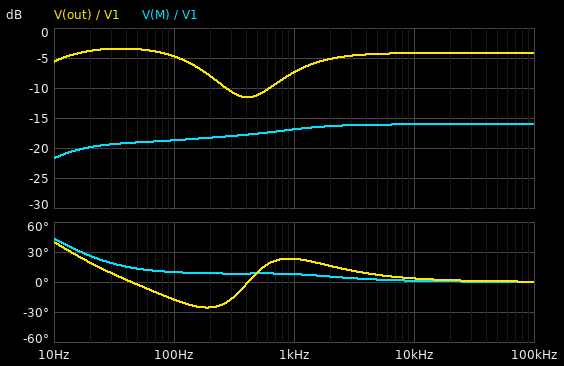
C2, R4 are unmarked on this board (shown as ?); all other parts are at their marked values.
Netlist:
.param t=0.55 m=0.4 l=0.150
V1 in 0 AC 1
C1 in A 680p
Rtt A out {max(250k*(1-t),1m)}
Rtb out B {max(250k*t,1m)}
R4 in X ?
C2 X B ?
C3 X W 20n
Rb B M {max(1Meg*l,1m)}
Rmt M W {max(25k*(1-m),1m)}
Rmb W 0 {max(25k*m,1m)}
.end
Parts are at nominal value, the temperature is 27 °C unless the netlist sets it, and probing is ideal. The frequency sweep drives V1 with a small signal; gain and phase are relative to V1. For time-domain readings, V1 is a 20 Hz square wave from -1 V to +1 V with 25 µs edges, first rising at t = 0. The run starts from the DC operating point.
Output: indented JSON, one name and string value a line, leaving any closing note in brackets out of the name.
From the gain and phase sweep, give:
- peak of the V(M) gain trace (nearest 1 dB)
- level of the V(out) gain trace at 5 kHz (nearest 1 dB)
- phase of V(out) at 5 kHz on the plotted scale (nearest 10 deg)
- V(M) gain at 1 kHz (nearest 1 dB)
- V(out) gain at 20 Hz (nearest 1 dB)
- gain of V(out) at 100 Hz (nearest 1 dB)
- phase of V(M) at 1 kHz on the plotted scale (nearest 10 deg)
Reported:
{
  "peak of the V(M) gain trace": "-16 dB",
  "level of the V(out) gain trace at 5 kHz": "-4 dB",
  "phase of V(out) at 5 kHz on the plotted scale": "10 deg",
  "V(M) gain at 1 kHz": "-17 dB",
  "V(out) gain at 20 Hz": "-4 dB",
  "gain of V(out) at 100 Hz": "-5 dB",
  "phase of V(M) at 1 kHz on the plotted scale": "10 deg"
}
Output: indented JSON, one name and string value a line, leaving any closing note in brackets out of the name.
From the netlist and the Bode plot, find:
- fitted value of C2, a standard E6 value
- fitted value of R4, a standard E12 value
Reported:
{
  "fitted value of C2, a standard E6 value": "68 nF",
  "fitted value of R4, a standard E12 value": "68 kΩ"
}
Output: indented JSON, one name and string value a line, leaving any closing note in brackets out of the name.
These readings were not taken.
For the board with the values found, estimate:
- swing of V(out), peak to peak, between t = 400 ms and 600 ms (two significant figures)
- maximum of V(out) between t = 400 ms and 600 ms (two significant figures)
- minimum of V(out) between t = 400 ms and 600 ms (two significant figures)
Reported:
{
  "swing of V(out), peak to peak, between t = 400 ms and 600 ms": "1.9 V",
  "maximum of V(out) between t = 400 ms and 600 ms": "950 mV",
  "minimum of V(out) between t = 400 ms and 600 ms": "-950 mV"
}
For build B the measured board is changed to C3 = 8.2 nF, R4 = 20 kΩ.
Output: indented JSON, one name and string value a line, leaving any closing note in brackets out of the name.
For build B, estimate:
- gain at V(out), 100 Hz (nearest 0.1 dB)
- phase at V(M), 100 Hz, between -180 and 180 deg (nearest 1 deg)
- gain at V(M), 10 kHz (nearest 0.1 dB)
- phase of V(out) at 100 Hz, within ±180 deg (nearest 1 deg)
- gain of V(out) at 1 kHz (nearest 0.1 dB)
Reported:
{
  "gain at V(out), 100 Hz": "-1.0 dB",
  "phase at V(M), 100 Hz, between -180 and 180 deg": "17 deg",
  "gain at V(M), 10 kHz": "-9.1 dB",
  "phase of V(out) at 100 Hz, within ±180 deg": "3 deg",
  "gain of V(out) at 1 kHz": "-4.1 dB"
}
